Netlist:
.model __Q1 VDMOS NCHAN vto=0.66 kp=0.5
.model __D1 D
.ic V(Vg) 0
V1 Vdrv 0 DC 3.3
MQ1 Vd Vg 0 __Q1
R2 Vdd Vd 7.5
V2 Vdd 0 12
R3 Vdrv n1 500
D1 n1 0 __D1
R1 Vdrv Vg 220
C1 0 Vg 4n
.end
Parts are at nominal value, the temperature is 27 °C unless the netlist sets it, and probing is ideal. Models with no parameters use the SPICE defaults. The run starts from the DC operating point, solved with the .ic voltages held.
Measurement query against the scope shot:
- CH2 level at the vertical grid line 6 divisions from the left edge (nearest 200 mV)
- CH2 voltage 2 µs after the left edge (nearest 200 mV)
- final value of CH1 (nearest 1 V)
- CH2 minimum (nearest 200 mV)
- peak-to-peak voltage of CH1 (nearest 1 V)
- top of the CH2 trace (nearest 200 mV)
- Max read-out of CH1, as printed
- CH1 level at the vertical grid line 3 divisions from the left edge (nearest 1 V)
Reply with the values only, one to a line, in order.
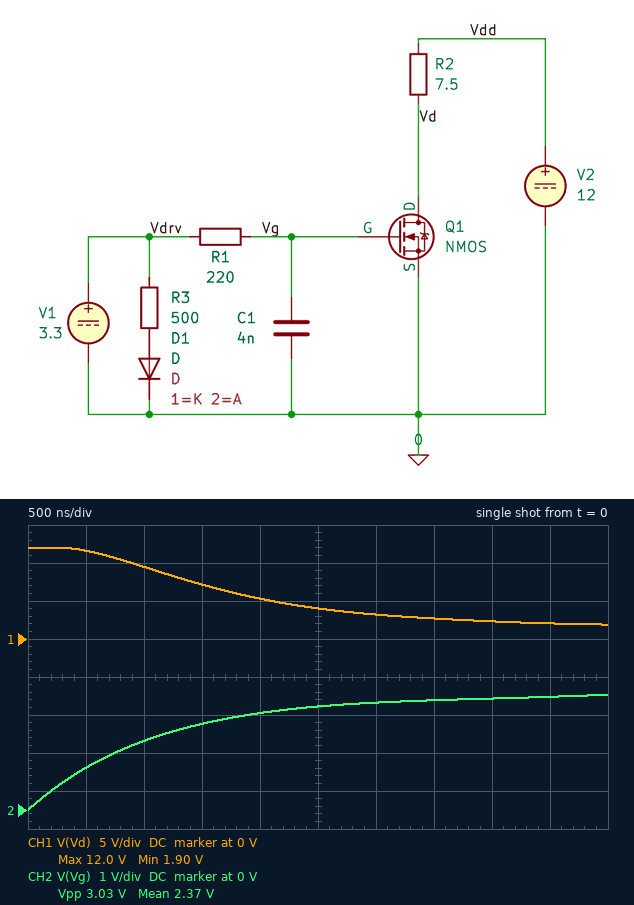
2.8 V
2.6 V
2 V
0 V
10 V
3.0 V
12.0 V
7 V
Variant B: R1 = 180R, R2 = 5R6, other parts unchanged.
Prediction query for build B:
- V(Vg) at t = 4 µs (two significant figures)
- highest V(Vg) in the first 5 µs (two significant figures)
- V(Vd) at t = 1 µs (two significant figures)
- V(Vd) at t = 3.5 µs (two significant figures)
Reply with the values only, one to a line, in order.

3.1 V
3.2 V
9.3 V
3.7 V
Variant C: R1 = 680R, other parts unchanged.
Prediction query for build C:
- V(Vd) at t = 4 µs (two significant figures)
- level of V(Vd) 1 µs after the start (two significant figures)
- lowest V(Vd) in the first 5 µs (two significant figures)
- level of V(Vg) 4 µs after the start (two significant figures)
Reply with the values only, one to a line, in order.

8.1 V
12 V
6.7 V
2.1 V
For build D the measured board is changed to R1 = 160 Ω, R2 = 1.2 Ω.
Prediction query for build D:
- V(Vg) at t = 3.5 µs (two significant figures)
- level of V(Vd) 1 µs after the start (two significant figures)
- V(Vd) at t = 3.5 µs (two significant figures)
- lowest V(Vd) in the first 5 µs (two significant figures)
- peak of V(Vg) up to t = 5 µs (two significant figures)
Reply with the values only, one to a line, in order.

3.2 V
11 V
10 V
9.9 V
3.3 V
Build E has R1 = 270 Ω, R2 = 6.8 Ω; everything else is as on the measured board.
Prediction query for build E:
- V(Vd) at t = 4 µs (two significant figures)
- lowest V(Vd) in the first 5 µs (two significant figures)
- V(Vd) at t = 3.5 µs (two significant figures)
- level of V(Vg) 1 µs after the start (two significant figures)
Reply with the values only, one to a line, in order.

3.4 V
2.8 V
4.0 V
1.6 V
